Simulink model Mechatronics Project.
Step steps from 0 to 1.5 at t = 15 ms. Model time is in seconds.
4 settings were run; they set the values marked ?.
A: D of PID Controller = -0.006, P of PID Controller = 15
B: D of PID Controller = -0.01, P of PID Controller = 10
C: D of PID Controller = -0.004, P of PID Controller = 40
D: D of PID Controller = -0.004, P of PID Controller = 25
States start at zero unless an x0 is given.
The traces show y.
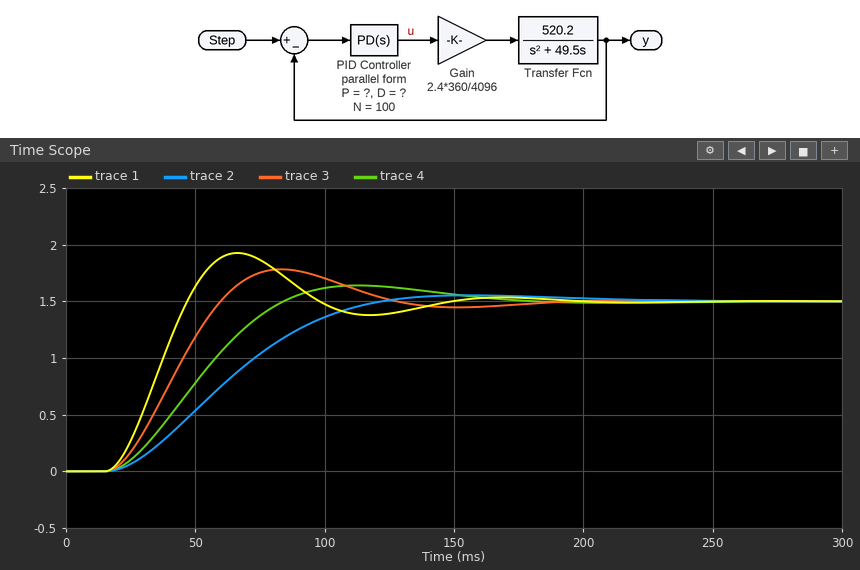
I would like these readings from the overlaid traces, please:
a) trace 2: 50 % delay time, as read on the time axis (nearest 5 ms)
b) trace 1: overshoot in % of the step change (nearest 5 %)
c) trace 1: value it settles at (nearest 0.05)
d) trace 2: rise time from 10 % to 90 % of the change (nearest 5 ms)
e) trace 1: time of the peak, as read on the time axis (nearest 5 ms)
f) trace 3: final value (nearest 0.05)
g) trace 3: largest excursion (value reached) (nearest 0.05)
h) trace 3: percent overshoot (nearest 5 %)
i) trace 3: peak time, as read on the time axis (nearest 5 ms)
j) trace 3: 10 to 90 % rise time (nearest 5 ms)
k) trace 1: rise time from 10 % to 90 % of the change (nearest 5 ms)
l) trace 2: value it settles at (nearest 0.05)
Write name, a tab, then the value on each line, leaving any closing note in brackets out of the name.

trace 2: 50 % delay time, as read on the time axis	60 ms
trace 1: overshoot in % of the step change	30 %
trace 1: value it settles at	1.50
trace 2: rise time from 10 % to 90 % of the change	70 ms
trace 1: time of the peak, as read on the time axis	65 ms
trace 3: final value	1.50
trace 3: largest excursion (value reached)	1.80
trace 3: percent overshoot	20 %
trace 3: peak time, as read on the time axis	85 ms
trace 3: 10 to 90 % rise time	30 ms
trace 1: rise time from 10 % to 90 % of the change	20 ms
trace 2: value it settles at	1.50
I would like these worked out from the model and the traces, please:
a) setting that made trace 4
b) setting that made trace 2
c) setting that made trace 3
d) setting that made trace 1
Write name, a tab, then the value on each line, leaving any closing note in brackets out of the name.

setting that made trace 4	A
setting that made trace 2	B
setting that made trace 3	D
setting that made trace 1	C
